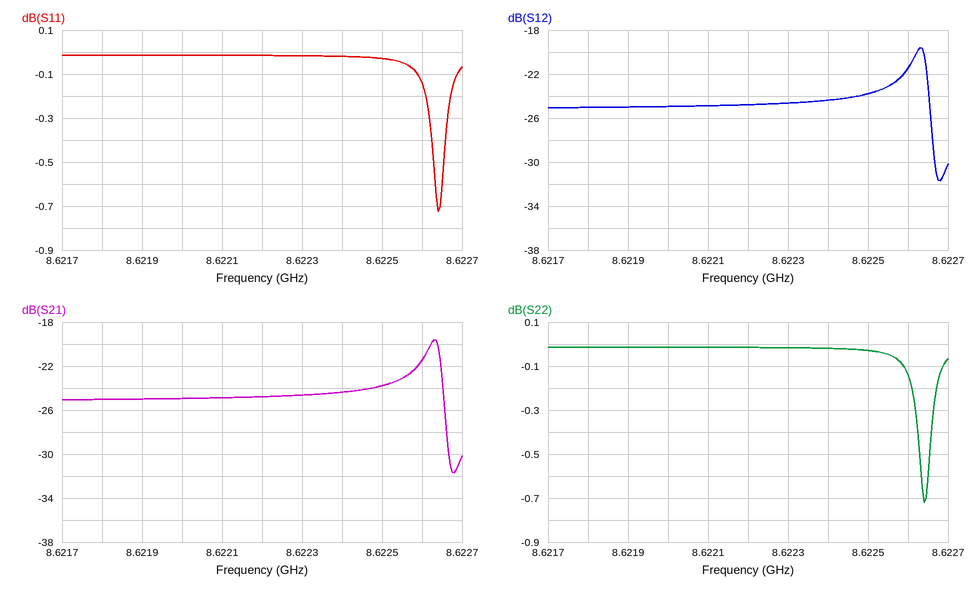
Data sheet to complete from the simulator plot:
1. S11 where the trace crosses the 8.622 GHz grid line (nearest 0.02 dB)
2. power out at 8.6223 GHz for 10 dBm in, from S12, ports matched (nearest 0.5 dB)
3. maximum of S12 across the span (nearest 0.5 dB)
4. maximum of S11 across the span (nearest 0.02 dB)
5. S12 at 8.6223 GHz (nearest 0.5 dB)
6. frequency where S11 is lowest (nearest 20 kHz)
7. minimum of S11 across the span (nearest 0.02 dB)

-0.02 dB
-14.5 dBm
-19.5 dB
-0.02 dB
-24.5 dB
8.62264 GHz
-0.72 dB
